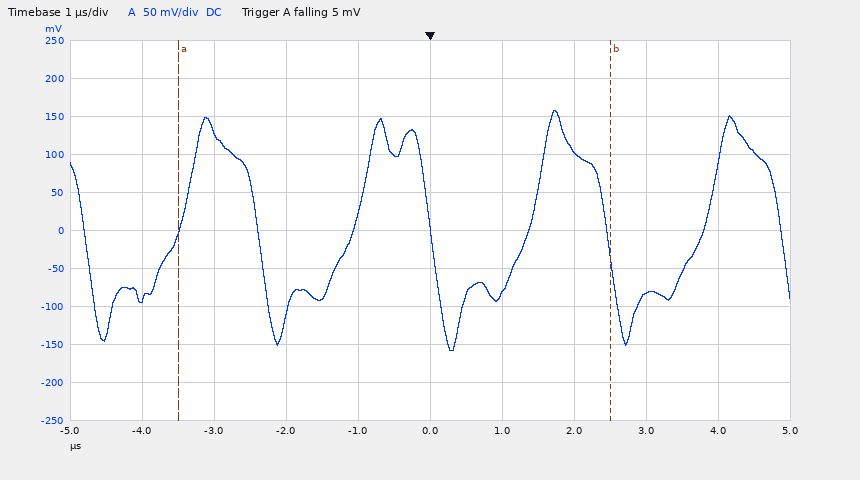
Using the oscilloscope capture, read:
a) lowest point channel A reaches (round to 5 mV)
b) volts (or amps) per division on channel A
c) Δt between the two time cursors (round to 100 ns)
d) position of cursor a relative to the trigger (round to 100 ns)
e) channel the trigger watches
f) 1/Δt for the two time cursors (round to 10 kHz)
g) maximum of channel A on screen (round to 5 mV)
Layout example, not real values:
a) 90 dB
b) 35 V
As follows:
a) -160 mV
b) 50 mV
c) 6.0 µs
d) -3.5 µs
e) channel A
f) 170 kHz
g) 160 mV
